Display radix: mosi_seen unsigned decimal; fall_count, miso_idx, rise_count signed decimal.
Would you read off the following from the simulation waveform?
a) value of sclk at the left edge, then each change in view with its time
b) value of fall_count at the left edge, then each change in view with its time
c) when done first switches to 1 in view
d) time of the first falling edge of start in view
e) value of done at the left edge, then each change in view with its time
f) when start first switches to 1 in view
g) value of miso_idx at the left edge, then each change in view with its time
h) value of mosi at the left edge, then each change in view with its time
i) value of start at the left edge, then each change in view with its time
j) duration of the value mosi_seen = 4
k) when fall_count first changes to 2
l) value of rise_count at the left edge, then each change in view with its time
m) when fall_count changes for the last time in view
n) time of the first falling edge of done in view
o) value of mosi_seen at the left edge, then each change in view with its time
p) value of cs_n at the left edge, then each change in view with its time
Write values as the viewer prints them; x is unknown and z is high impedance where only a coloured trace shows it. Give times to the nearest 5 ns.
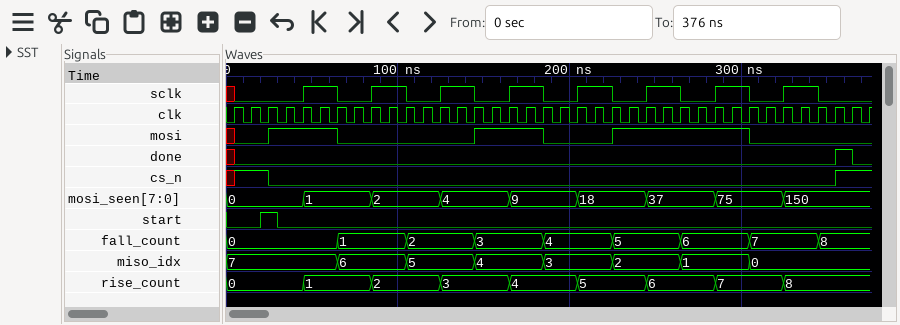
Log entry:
x, 0 at 5 ns, 1 at 45 ns, 0 at 65 ns, 1 at 85 ns, 0 at 105 ns, 1 at 125 ns, 0 at 145 ns, 1 at 165 ns, 0 at 185 ns, 1 at 205 ns, 0 at 225 ns, 1 at 245 ns, 0 at 265 ns, 1 at 285 ns, 0 at 305 ns, 1 at 325 ns, 0 at 345 ns
0, 1 at 65 ns, 2 at 105 ns, 3 at 145 ns, 4 at 185 ns, 5 at 225 ns, 6 at 265 ns, 7 at 305 ns, 8 at 345 ns
355 ns
30 ns
x, 0 at 5 ns, 1 at 355 ns, 0 at 365 ns
20 ns
7, 6 at 65 ns, 5 at 105 ns, 4 at 145 ns, 3 at 185 ns, 2 at 225 ns, 1 at 265 ns, 0 at 305 ns
x, 0 at 5 ns, 1 at 25 ns, 0 at 65 ns, 1 at 145 ns, 0 at 185 ns, 1 at 225 ns, 0 at 305 ns
0, 1 at 20 ns, 0 at 30 ns
40 ns
105 ns
0, 1 at 45 ns, 2 at 85 ns, 3 at 125 ns, 4 at 165 ns, 5 at 205 ns, 6 at 245 ns, 7 at 285 ns, 8 at 325 ns
345 ns
365 ns
0, 1 at 45 ns, 2 at 85 ns, 4 at 125 ns, 9 at 165 ns, 18 at 205 ns, 37 at 245 ns, 75 at 285 ns, 150 at 325 ns
x, 1 at 5 ns, 0 at 25 ns, 1 at 355 ns
